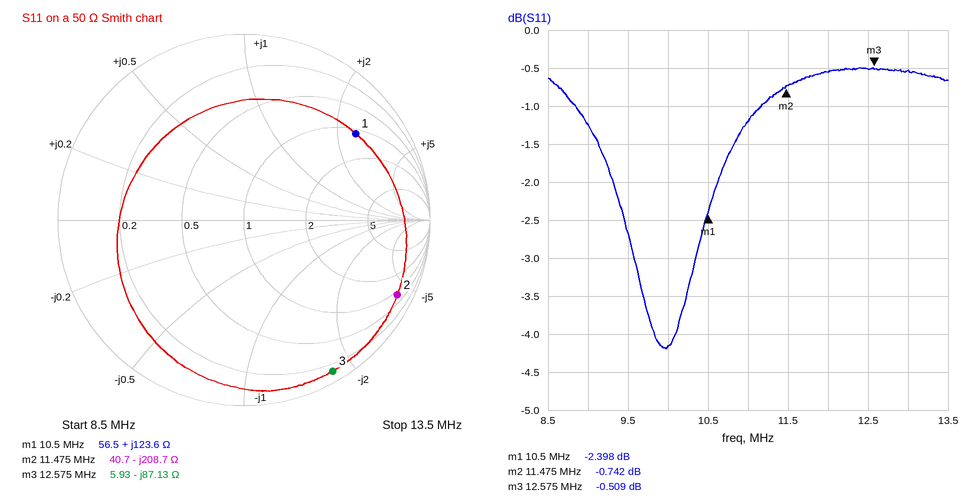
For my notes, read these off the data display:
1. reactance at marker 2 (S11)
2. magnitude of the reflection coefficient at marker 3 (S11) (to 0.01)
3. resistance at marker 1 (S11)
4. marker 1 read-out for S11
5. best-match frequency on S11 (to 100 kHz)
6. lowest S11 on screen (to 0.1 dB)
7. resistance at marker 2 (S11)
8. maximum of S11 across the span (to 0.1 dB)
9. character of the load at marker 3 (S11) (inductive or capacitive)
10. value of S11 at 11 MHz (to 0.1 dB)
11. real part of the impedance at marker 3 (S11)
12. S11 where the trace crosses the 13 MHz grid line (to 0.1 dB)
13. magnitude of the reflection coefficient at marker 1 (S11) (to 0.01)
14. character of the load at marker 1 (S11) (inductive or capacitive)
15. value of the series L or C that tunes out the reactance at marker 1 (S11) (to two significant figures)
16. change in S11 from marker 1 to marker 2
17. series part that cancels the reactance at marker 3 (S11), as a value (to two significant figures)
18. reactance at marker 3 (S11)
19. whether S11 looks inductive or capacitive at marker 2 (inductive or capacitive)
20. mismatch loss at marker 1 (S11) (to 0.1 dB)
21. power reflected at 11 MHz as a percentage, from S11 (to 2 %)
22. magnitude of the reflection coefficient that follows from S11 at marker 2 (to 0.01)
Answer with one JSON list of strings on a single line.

["-208.7 Ω", "0.94", "56.5 Ω", "-2.398 dB", "10.0 MHz", "-4.2 dB", "40.7 Ω", "-0.5 dB", "capacitive", "-1.2 dB", "5.93 Ω", "-0.5 dB", "0.76", "inductive", "120 pF", "1.656 dB", "1.1 µH", "-87.13 Ω", "capacitive", "3.7 dB", "76 %", "0.92"]
